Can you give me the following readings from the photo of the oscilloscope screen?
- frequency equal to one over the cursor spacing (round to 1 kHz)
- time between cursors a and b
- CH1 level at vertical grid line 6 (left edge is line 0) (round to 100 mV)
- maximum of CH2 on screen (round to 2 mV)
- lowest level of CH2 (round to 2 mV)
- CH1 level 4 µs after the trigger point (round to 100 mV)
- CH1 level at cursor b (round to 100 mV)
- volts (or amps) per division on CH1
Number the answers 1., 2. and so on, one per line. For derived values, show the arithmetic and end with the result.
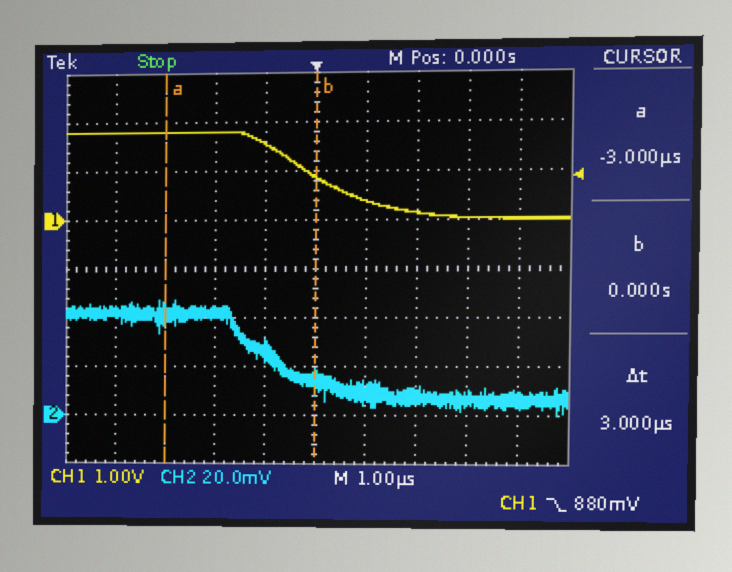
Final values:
1. 1 / 3 µs ≈ 333 kHz
2. 3 µs
3. 400 mV
4. 48 mV
5. 0 mV
6. 0.0 V
7. 900 mV
8. 1 V
